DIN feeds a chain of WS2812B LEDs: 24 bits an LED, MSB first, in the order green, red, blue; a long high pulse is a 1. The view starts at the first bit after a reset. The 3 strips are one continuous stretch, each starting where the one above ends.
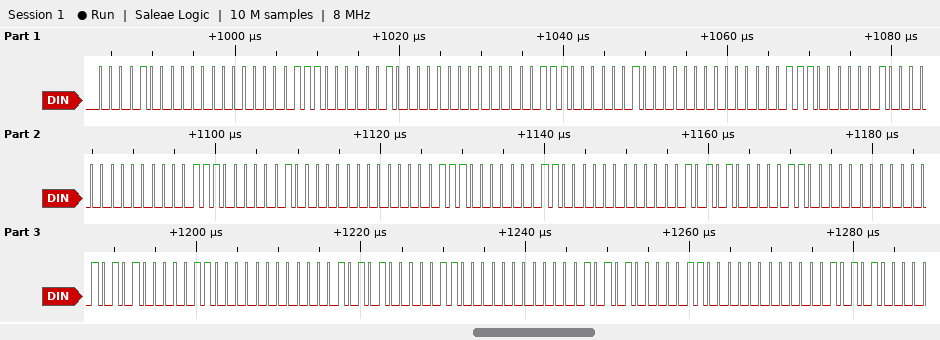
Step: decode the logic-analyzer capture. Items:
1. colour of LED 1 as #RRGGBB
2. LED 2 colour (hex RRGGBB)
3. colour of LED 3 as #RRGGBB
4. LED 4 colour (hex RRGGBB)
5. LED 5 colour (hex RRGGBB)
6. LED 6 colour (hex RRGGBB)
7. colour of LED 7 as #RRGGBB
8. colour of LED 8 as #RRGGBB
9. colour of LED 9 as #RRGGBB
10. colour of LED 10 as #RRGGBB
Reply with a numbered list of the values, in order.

1. #00081C
2. #00081C
3. #00081C
4. #00081C
5. #00081C
6. #000615
7. #000615
8. #000615
9. #000615
10. #000615
